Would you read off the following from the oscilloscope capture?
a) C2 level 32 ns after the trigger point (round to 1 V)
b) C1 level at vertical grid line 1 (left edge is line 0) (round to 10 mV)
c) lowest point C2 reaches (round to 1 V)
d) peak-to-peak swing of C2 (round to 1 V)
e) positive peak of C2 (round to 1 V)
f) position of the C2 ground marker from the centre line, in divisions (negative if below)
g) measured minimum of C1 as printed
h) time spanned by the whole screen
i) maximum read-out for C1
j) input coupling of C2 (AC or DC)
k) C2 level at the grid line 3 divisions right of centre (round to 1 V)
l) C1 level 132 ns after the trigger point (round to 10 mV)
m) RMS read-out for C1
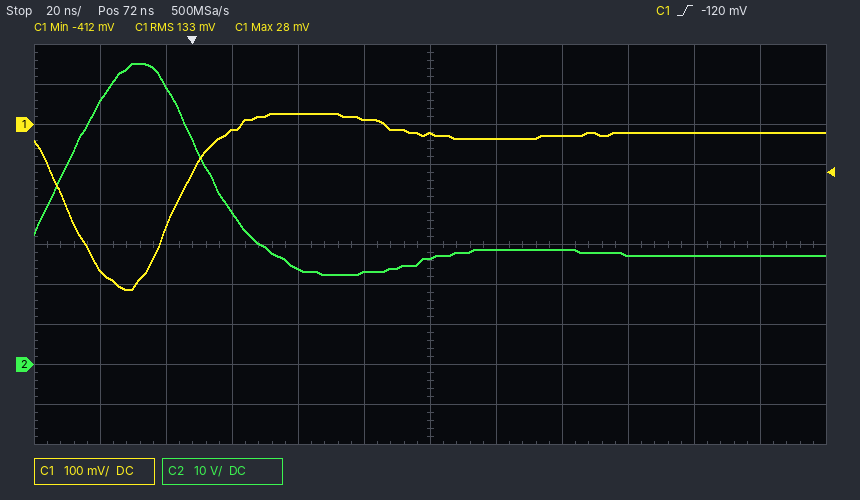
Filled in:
24 V
-360 mV
22 V
53 V
75 V
-3.0 div
-412 mV
240 ns
28 mV
DC
27 V
-20 mV
133 mV
